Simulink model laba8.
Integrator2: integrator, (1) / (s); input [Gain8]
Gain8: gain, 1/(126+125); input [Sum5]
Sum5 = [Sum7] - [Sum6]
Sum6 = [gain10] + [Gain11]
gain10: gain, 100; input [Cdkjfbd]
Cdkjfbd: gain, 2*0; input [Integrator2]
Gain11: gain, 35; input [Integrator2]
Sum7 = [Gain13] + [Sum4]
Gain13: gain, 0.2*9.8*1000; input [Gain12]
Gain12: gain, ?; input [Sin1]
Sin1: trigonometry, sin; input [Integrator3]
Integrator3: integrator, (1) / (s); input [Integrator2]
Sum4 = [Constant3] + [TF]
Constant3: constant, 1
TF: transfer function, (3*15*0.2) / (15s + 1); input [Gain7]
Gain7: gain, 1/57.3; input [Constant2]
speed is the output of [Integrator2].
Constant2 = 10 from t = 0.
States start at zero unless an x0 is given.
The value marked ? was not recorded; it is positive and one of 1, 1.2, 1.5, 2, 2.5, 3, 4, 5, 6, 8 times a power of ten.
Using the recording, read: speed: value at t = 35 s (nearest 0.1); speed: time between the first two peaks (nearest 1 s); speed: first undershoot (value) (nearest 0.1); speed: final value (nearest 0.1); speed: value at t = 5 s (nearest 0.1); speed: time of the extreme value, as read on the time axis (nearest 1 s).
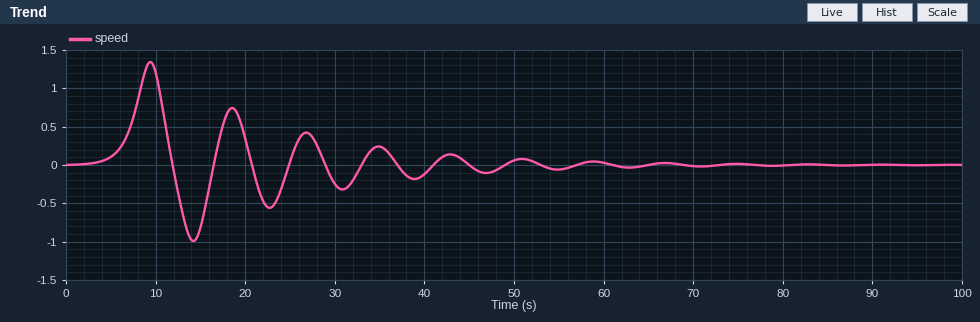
0.2
9 s
-1.0
0.0
0.1
9 s
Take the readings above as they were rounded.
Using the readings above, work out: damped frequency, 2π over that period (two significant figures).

0.70 rad/s
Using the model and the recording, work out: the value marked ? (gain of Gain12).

0.08
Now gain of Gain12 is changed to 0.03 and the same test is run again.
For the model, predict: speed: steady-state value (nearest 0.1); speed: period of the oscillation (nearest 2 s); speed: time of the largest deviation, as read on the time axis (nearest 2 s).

0.0
14 s
14 s
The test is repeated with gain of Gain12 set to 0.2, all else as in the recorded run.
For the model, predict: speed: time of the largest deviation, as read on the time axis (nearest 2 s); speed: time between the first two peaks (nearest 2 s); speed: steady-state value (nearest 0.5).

6 s
6 s
0.0
